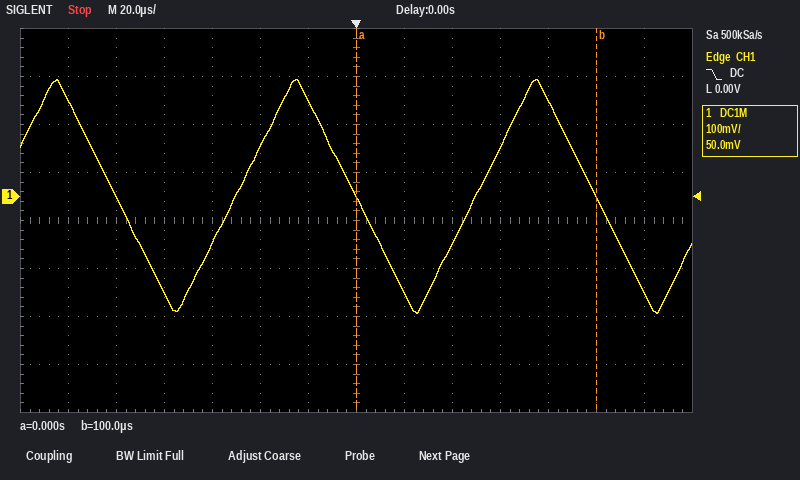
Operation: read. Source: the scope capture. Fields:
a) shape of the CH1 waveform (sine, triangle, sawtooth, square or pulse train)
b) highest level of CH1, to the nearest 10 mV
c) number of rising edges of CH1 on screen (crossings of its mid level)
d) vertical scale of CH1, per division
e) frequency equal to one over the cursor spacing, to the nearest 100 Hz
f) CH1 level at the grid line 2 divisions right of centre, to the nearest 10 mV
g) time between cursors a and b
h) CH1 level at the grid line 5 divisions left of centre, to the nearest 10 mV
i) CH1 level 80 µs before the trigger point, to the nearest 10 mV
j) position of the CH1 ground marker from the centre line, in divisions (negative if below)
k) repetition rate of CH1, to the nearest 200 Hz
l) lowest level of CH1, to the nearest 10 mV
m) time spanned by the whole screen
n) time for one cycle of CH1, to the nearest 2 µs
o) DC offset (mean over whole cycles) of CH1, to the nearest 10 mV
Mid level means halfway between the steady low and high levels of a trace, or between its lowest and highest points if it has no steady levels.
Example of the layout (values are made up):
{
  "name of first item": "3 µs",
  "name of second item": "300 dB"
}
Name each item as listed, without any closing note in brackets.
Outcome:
{
  "shape of the CH1 waveform": "triangle",
  "highest level of CH1, to the nearest 10 mV": "240 mV",
  "number of rising edges of CH1 on screen": "2",
  "vertical scale of CH1, per division": "100 mV",
  "frequency equal to one over the cursor spacing, to the nearest 100 Hz": "10.0 kHz",
  "CH1 level at the grid line 2 divisions right of centre, to the nearest 10 mV": "-100 mV",
  "time between cursors a and b": "100 µs",
  "CH1 level at the grid line 5 divisions left of centre, to the nearest 10 mV": "0 mV",
  "CH1 level 80 µs before the trigger point, to the nearest 10 mV": "-200 mV",
  "position of the CH1 ground marker from the centre line, in divisions": "+0.5 div",
  "repetition rate of CH1, to the nearest 200 Hz": "10.0 kHz",
  "lowest level of CH1, to the nearest 10 mV": "-240 mV",
  "time spanned by the whole screen": "280 µs",
  "time for one cycle of CH1, to the nearest 2 µs": "100 µs",
  "DC offset (mean over whole cycles) of CH1, to the nearest 10 mV": "0 mV"
}
